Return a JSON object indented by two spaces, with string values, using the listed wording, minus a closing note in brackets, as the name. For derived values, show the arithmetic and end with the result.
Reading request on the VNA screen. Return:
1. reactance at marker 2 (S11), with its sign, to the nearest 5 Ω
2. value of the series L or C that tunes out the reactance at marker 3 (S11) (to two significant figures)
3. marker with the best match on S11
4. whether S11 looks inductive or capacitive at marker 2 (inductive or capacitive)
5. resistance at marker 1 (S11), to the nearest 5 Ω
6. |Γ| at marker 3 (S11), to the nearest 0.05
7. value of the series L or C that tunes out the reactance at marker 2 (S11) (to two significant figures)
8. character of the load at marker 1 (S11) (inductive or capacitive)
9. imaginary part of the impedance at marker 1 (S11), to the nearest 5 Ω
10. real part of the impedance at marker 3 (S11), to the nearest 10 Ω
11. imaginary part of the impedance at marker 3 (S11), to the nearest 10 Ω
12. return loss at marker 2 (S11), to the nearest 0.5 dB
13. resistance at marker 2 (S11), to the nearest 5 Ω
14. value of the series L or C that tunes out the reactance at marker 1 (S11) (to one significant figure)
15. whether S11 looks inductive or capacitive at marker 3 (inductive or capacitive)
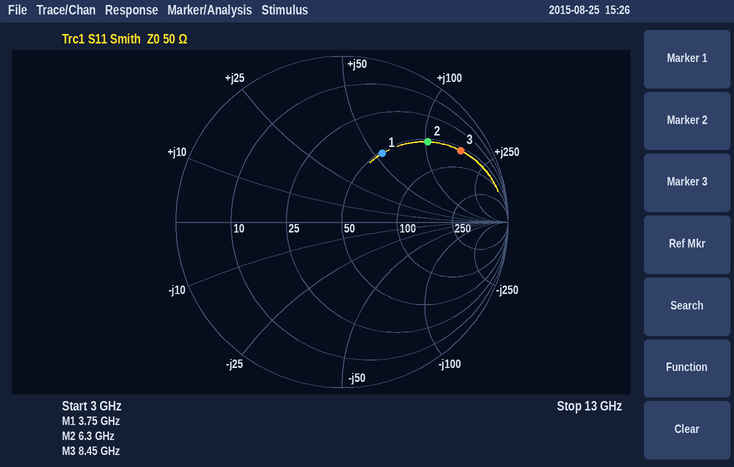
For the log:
{
  "reactance at marker 2 (S11), with its sign, to the nearest 5 Ω": "+105 Ω",
  "value of the series L or C that tunes out the reactance at marker 3 (S11)": "C = 1/(2π × 8.45 GHz × 160 Ω) ≈ 118 fF, so 120 fF to two significant figures",
  "marker with the best match on S11": "marker 1",
  "whether S11 looks inductive or capacitive at marker 2": "inductive",
  "resistance at marker 1 (S11), to the nearest 5 Ω": "50 Ω",
  "|Γ| at marker 3 (S11), to the nearest 0.05": "0.85",
  "value of the series L or C that tunes out the reactance at marker 2 (S11)": "C = 1/(2π × 6.3 GHz × 105 Ω) ≈ 241 fF, so 240 fF to two significant figures",
  "character of the load at marker 1 (S11)": "inductive",
  "imaginary part of the impedance at marker 1 (S11), to the nearest 5 Ω": "+55 Ω",
  "real part of the impedance at marker 3 (S11), to the nearest 10 Ω": "60 Ω",
  "imaginary part of the impedance at marker 3 (S11), to the nearest 10 Ω": "+160 Ω",
  "return loss at marker 2 (S11), to the nearest 0.5 dB": "3.0 dB",
  "resistance at marker 2 (S11), to the nearest 5 Ω": "55 Ω",
  "value of the series L or C that tunes out the reactance at marker 1 (S11)": "C = 1/(2π × 3.75 GHz × 55 Ω) ≈ 772 fF, so 800 fF to one significant figure",
  "whether S11 looks inductive or capacitive at marker 3": "inductive"
}
